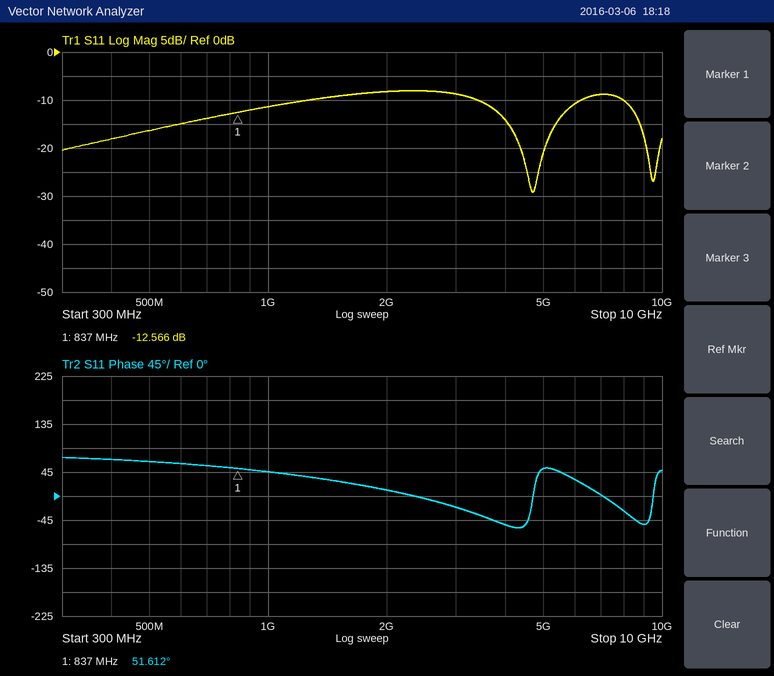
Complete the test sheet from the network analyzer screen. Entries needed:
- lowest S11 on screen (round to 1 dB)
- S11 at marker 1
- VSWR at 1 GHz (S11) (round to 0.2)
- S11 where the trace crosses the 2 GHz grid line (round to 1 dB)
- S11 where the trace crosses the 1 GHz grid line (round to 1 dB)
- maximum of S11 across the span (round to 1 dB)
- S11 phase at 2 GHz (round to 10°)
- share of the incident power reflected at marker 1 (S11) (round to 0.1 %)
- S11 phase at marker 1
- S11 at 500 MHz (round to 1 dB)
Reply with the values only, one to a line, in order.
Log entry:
-29 dB
-12.566 dB
1.8
-8 dB
-11 dB
-8 dB
10°
5.5 %
51.612°
-16 dB
